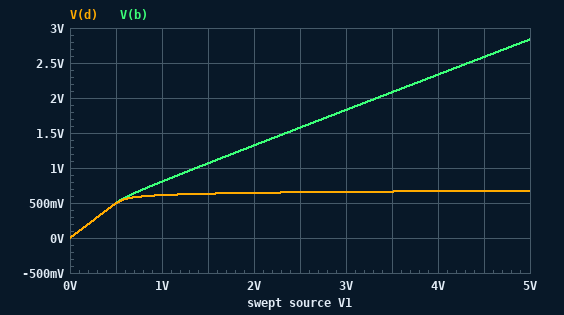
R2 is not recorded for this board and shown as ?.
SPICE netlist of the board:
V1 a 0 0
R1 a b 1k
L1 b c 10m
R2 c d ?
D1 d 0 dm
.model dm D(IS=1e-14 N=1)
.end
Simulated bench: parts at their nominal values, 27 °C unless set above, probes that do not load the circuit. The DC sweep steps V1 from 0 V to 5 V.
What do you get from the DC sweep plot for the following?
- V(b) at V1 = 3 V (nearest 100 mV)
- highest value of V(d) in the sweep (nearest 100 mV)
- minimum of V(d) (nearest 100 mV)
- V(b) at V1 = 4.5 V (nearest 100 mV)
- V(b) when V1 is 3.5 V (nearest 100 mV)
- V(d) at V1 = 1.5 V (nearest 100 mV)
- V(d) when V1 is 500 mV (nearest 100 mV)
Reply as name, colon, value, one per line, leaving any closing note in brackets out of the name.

V(b) at V1 = 3 V: 1.8 V
highest value of V(d) in the sweep: 700 mV
minimum of V(d): 0 V
V(b) at V1 = 4.5 V: 2.6 V
V(b) when V1 is 3.5 V: 2.1 V
V(d) at V1 = 1.5 V: 600 mV
V(d) when V1 is 500 mV: 500 mV
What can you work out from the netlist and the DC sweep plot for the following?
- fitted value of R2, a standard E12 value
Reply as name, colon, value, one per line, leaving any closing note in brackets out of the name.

fitted value of R2, a standard E12 value: 1 kΩ
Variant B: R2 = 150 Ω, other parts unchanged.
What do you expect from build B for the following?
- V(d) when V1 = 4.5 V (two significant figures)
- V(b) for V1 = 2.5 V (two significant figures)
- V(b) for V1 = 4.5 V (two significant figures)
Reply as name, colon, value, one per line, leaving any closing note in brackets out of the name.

V(d) when V1 = 4.5 V: 690 mV
V(b) for V1 = 2.5 V: 910 mV
V(b) for V1 = 4.5 V: 1.2 V
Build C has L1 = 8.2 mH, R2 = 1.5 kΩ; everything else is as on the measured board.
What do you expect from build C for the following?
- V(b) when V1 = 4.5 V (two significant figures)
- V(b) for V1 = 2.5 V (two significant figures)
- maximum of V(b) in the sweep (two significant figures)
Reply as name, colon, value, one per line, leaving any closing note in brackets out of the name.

V(b) when V1 = 4.5 V: 3.0 V
V(b) for V1 = 2.5 V: 1.8 V
maximum of V(b) in the sweep: 3.3 V
